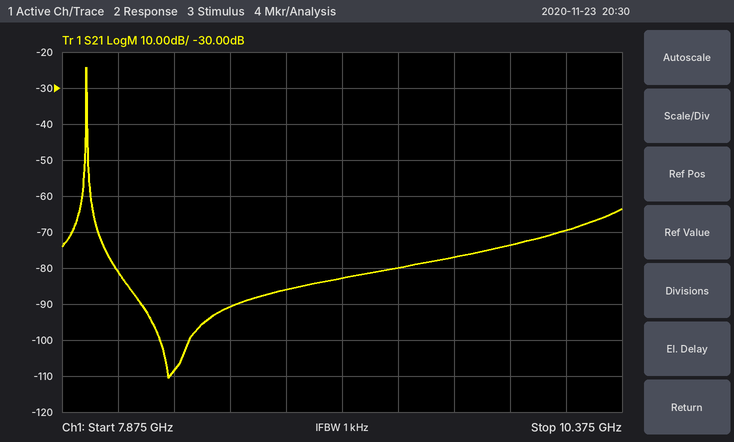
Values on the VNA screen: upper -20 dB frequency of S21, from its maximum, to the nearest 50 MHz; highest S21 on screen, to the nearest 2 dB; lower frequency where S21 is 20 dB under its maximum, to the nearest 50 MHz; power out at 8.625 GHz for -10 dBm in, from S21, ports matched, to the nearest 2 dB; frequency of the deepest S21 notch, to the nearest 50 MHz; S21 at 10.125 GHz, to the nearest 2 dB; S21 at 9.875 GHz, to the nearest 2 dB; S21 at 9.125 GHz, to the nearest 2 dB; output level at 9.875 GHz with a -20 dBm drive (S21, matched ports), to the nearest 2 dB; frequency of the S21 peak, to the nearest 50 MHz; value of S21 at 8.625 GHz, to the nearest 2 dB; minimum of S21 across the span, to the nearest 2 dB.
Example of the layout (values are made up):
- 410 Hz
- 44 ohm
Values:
- 8.00 GHz
- -24 dB
- 8.00 GHz
- -100 dBm
- 8.35 GHz
- -70 dB
- -74 dB
- -82 dB
- -94 dBm
- 8.00 GHz
- -90 dB
- -110 dB
